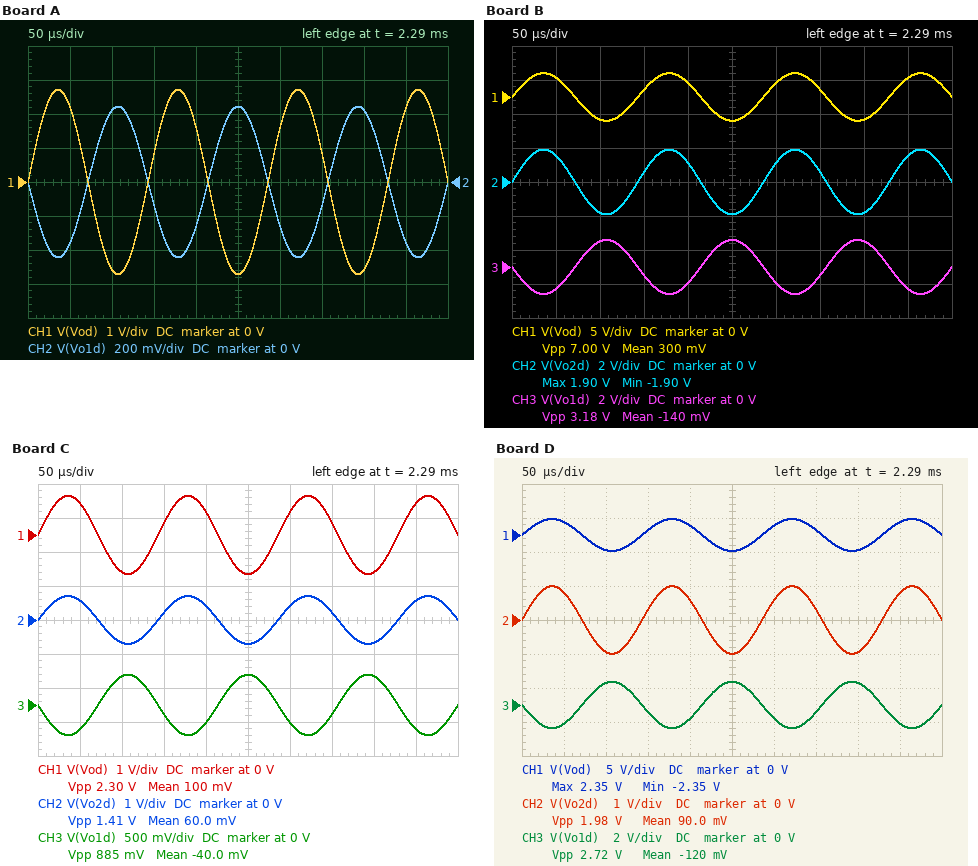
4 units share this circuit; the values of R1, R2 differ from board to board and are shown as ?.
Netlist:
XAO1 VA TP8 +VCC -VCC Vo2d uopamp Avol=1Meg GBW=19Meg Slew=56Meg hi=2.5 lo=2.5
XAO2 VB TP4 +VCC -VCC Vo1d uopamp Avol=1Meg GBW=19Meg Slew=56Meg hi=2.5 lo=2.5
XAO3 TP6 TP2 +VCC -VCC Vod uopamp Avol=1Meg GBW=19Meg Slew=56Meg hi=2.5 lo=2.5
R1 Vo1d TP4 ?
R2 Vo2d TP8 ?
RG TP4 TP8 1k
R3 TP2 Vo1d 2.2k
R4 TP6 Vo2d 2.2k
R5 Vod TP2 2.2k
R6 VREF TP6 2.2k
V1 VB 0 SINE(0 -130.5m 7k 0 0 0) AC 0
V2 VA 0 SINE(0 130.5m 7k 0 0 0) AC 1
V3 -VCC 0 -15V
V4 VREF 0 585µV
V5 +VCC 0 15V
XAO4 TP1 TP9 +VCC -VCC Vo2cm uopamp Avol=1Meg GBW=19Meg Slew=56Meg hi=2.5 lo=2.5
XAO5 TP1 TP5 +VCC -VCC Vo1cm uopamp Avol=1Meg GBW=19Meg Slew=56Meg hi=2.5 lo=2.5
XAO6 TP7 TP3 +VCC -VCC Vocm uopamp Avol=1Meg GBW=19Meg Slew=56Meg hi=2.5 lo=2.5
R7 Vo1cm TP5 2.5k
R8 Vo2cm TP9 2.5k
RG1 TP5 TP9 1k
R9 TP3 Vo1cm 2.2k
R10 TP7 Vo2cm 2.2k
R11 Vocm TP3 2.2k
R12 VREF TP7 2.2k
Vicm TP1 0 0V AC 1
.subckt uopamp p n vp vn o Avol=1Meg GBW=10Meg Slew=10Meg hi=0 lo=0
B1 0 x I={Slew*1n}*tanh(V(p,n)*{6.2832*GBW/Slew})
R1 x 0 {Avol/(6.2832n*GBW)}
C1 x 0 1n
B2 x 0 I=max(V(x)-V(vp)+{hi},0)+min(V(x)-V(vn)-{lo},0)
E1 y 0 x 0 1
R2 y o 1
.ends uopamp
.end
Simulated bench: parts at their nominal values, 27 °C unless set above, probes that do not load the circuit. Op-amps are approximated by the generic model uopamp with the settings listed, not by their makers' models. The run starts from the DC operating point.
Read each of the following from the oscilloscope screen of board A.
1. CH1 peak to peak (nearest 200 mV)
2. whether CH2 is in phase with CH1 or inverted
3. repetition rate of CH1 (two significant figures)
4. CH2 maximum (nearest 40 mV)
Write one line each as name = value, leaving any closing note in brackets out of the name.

CH1 peak to peak = 5.4 V
whether CH2 is in phase with CH1 or inverted = inverted
repetition rate of CH1 = 7.0 kHz
CH2 maximum = 440 mV
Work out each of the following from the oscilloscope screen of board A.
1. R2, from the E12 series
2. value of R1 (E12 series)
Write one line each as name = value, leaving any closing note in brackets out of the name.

R2, from the E12 series = 8.2 kΩ
value of R1 = 1.2 kΩ
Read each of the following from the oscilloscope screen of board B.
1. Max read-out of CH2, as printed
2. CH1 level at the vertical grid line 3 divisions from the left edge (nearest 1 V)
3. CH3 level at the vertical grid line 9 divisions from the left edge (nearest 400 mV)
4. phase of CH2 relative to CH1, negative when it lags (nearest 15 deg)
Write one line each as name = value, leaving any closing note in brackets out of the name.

Max read-out of CH2, as printed = 1.90 V
CH1 level at the vertical grid line 3 divisions from the left edge = 1 V
CH3 level at the vertical grid line 9 divisions from the left edge = -1.2 V
phase of CH2 relative to CH1, negative when it lags = 0 deg
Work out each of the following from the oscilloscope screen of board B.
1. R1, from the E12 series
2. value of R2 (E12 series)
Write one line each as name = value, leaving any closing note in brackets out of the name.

R1, from the E12 series = 5.6 kΩ
value of R2 = 6.8 kΩ
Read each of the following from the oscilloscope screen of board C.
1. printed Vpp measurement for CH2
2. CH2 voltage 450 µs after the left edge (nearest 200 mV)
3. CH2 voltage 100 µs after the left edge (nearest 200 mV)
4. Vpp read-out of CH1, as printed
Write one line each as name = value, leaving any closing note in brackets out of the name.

printed Vpp measurement for CH2 = 1.41 V
CH2 voltage 450 µs after the left edge = 600 mV
CH2 voltage 100 µs after the left edge = -600 mV
Vpp read-out of CH1, as printed = 2.30 V
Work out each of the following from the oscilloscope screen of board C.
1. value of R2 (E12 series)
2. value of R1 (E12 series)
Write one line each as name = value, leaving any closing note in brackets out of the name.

value of R2 = 2.2 kΩ
value of R1 = 1.2 kΩ
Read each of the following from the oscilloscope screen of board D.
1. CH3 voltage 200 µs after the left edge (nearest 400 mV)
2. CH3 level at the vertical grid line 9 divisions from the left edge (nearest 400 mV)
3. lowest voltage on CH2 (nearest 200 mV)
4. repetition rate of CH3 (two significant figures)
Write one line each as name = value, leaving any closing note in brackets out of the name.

CH3 voltage 200 µs after the left edge = -800 mV
CH3 level at the vertical grid line 9 divisions from the left edge = -1.2 V
lowest voltage on CH2 = -1.0 V
repetition rate of CH3 = 7.0 kHz
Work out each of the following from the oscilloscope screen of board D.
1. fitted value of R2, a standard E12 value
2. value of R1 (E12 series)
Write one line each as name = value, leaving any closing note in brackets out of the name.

fitted value of R2, a standard E12 value = 3.3 kΩ
value of R1 = 4.7 kΩ
